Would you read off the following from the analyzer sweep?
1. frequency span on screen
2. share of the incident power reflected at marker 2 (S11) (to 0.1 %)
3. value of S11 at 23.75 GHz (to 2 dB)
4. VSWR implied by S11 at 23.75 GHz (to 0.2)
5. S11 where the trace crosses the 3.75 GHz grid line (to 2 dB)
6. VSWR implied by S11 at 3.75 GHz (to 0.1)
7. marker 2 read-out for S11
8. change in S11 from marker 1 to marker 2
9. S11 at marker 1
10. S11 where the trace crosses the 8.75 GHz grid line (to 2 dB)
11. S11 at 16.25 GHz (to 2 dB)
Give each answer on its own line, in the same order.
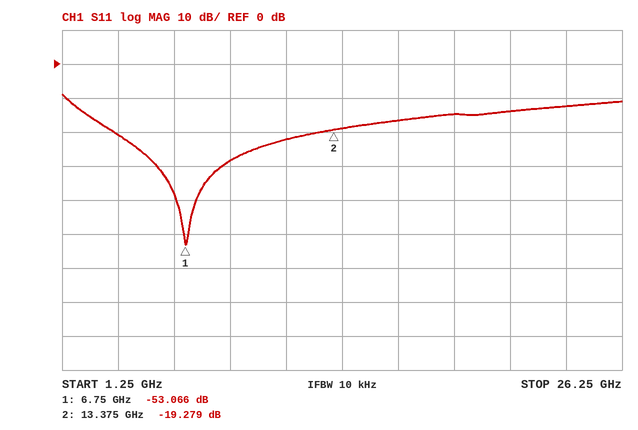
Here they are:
25 GHz
1.2 %
-12 dB
1.6
-20 dB
1.2
-19.279 dB
33.787 dB
-53.066 dB
-28 dB
-16 dB
